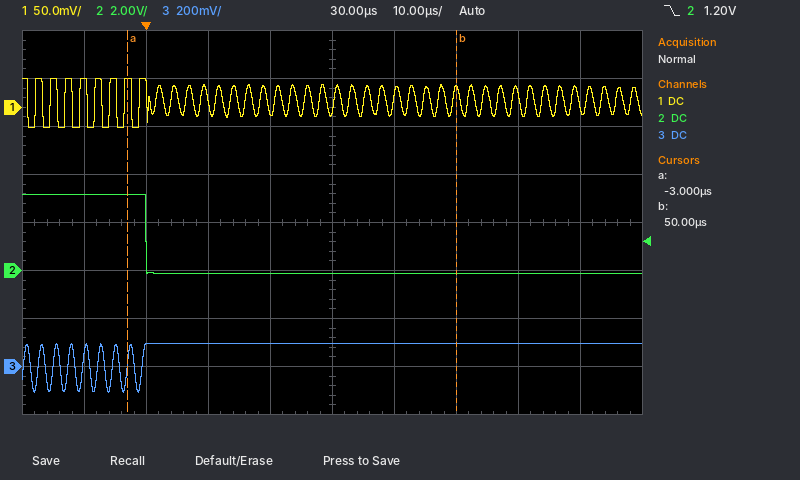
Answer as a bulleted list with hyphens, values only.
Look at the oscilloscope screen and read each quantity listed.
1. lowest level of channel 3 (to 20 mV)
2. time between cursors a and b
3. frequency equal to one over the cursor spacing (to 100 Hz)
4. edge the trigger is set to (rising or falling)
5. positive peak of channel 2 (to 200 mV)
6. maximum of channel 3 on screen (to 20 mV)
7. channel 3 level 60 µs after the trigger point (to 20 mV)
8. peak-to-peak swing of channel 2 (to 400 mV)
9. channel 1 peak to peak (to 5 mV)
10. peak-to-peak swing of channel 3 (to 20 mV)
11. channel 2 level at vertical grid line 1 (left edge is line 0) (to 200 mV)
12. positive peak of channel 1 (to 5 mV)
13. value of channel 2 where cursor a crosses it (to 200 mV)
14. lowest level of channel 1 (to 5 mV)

- -100 mV
- 53 µs
- 18.9 kHz
- falling
- 3.2 V
- 100 mV
- 100 mV
- 3.2 V
- 50 mV
- 200 mV
- 3.2 V
- 30 mV
- 3.2 V
- -20 mV
